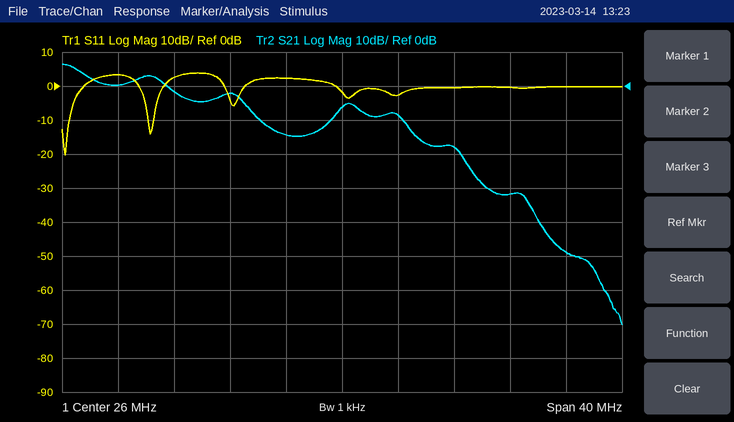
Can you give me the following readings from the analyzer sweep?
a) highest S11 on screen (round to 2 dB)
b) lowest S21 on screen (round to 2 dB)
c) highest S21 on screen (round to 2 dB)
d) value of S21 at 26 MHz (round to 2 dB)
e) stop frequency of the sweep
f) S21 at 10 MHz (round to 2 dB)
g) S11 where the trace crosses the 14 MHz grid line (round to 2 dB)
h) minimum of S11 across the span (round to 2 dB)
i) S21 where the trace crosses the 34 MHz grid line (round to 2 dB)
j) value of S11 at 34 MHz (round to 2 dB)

4 dB
-70 dB
6 dB
-6 dB
46 MHz
0 dB
2 dB
-20 dB
-18 dB
0 dB
